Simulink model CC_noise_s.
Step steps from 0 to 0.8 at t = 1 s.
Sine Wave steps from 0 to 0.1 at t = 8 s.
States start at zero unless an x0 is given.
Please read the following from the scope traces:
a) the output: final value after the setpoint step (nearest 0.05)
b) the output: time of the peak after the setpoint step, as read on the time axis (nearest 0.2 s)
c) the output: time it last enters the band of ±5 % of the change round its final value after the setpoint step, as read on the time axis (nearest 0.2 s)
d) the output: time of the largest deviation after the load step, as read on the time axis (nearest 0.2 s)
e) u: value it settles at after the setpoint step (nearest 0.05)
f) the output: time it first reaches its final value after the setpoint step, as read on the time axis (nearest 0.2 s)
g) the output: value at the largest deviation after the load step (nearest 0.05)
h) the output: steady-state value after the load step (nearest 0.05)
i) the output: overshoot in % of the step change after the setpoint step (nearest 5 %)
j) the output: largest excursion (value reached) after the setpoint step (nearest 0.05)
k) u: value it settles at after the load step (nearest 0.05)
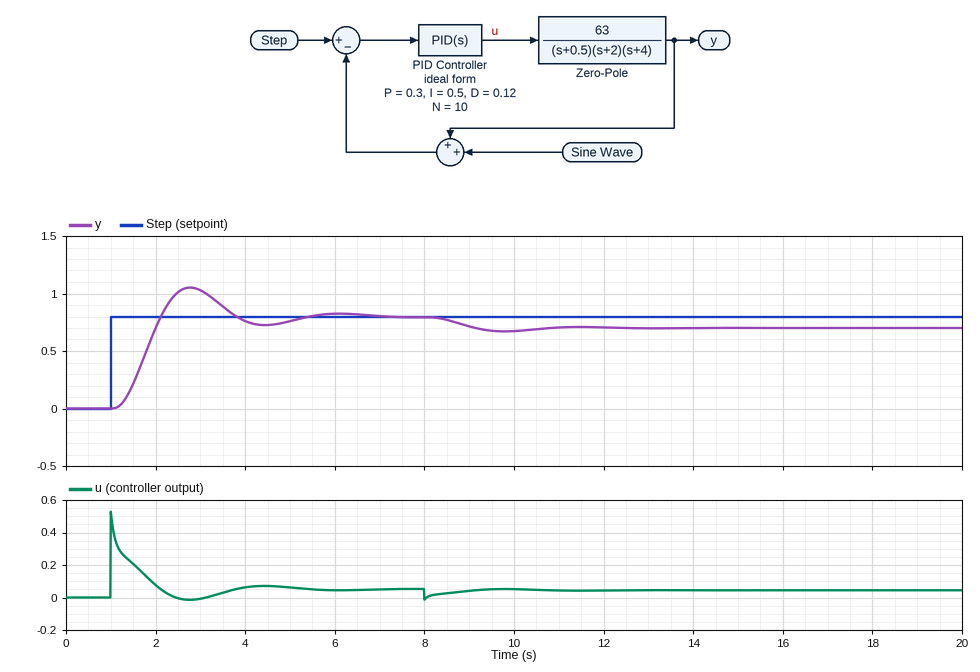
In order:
0.80
2.8 s
5.0 s
9.8 s
0.05
2.2 s
0.65
0.70
30 %
1.05
0.05
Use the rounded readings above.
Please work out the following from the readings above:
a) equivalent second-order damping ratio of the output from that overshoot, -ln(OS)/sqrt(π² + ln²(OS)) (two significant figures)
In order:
0.36
